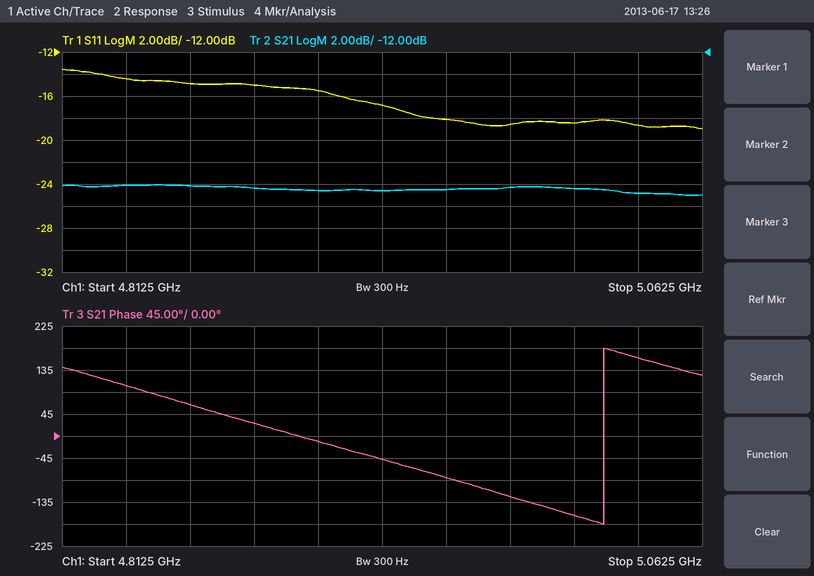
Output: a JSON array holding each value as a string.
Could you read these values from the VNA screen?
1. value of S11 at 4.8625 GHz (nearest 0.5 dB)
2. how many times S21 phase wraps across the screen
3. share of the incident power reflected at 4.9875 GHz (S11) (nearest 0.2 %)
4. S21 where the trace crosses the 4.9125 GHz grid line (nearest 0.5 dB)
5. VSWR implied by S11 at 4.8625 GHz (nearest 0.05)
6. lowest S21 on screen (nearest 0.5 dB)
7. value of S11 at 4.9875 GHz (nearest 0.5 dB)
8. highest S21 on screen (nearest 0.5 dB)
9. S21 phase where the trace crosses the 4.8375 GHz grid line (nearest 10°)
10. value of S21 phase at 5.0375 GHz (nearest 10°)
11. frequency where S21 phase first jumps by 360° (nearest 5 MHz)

["-15.0 dB", "1", "1.4 %", "-24.5 dB", "1.45", "-25.0 dB", "-18.5 dB", "-24.0 dB", "100°", "160°", "5.025 GHz"]
